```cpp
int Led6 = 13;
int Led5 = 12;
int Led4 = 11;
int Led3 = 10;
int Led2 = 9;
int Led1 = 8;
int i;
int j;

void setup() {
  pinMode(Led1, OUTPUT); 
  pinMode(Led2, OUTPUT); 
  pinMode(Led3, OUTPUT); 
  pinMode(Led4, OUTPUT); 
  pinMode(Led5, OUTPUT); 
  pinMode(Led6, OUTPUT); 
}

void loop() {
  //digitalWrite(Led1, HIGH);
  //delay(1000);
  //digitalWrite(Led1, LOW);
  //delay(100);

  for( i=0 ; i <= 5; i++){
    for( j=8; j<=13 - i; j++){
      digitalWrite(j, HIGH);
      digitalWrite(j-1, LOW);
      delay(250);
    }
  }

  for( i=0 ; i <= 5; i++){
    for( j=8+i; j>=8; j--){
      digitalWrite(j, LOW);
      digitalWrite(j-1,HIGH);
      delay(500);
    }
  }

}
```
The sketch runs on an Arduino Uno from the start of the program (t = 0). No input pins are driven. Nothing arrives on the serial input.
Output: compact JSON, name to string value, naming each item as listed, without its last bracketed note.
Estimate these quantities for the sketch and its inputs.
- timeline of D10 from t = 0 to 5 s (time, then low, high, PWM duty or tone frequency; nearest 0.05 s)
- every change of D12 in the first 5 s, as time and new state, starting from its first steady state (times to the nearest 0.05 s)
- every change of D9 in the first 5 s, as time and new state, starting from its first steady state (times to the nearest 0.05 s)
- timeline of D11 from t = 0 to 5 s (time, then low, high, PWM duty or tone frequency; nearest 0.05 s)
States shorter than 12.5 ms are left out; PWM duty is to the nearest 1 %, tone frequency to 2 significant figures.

{"timeline of D10 from t = 0 to 5 s": "0 s low; 0.5 s high; 0.75 s low; 2 s high; 2.25 s low; 3.25 s high; 3.5 s low; 4.25 s high", "every change of D12 in the first 5 s, as time and new state, starting from its first steady state": "0 s low; 1 s high; 1.25 s low; 2.5 s high", "every change of D9 in the first 5 s, as time and new state, starting from its first steady state": "0 s low; 0.25 s high; 0.5 s low; 1.75 s high; 2 s low; 3 s high; 3.25 s low; 4 s high; 4.25 s low; 4.75 s high", "timeline of D11 from t = 0 to 5 s": "0 s low; 0.75 s high; 1 s low; 2.25 s high; 2.5 s low; 3.5 s high"}
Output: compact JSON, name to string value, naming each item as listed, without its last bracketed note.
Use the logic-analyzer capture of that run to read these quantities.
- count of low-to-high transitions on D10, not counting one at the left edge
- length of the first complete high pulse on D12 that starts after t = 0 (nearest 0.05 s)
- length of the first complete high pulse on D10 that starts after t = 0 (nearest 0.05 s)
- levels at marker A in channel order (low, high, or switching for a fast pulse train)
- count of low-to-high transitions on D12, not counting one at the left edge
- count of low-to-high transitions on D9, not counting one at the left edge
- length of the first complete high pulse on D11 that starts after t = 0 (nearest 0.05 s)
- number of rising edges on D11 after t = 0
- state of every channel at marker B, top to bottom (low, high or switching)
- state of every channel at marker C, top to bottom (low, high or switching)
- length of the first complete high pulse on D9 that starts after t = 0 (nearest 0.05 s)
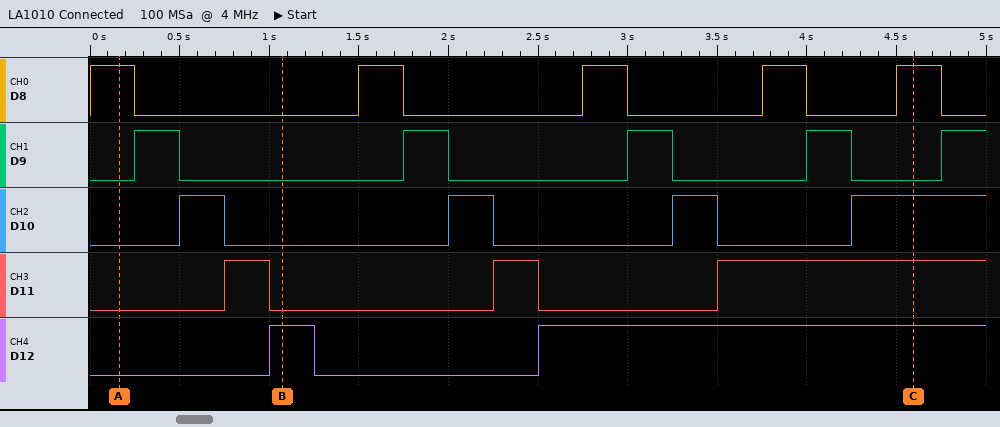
{"count of low-to-high transitions on D10, not counting one at the left edge": "4", "length of the first complete high pulse on D12 that starts after t = 0": "0.25 s", "length of the first complete high pulse on D10 that starts after t = 0": "0.25 s", "levels at marker A in channel order": "D8 high, D9 low, D10 low, D11 low, D12 low", "count of low-to-high transitions on D12, not counting one at the left edge": "2", "count of low-to-high transitions on D9, not counting one at the left edge": "5", "length of the first complete high pulse on D11 that starts after t = 0": "0.25 s", "number of rising edges on D11 after t = 0": "3", "state of every channel at marker B, top to bottom": "D8 low, D9 low, D10 low, D11 low, D12 high", "state of every channel at marker C, top to bottom": "D8 high, D9 low, D10 high, D11 high, D12 high", "length of the first complete high pulse on D9 that starts after t = 0": "0.25 s"}
